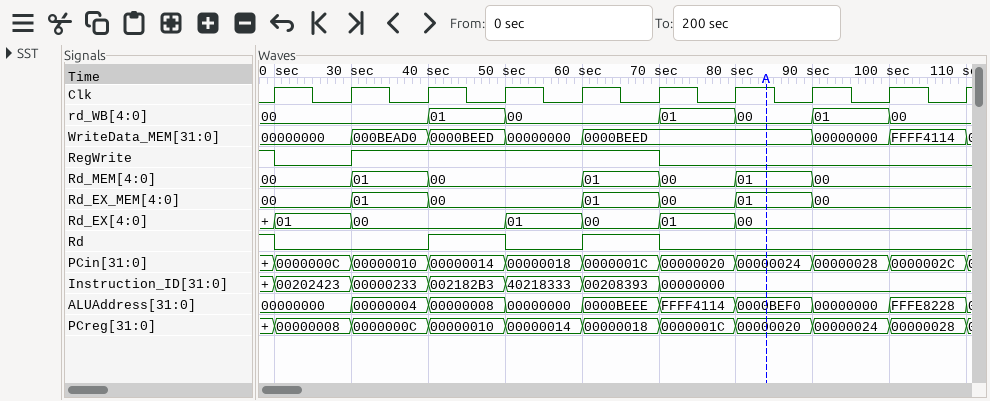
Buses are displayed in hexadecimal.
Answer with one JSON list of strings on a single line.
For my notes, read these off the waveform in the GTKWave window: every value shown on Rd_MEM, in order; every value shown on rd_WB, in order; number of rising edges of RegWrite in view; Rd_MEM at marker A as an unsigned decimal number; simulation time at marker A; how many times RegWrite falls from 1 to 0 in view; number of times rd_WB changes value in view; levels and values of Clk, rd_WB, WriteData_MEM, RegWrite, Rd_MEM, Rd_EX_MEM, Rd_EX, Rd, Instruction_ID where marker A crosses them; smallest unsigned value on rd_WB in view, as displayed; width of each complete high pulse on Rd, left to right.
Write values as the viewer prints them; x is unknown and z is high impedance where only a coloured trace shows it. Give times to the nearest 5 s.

["00, 01, 00, 01, 00, 01, 00", "00, 01, 00, 01, 00, 01, 00", "1", "1", "85 s", "2", "6", "Clk=1, rd_WB=00, WriteData_MEM=0000BEED, RegWrite=0, Rd_MEM=01, Rd_EX_MEM=01, Rd_EX=00, Rd=0, Instruction_ID=00000000", "00", "10 s, 10 s"]
